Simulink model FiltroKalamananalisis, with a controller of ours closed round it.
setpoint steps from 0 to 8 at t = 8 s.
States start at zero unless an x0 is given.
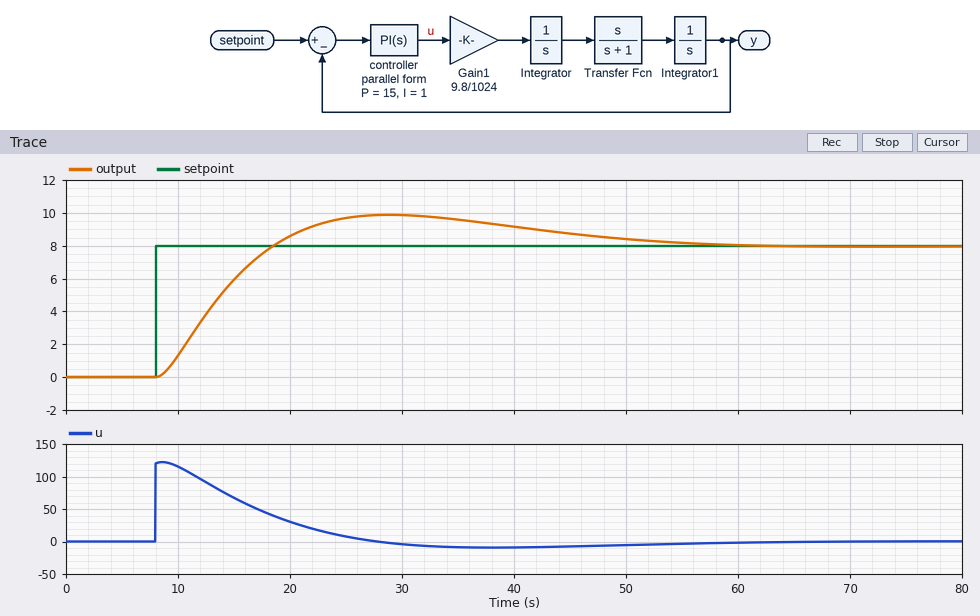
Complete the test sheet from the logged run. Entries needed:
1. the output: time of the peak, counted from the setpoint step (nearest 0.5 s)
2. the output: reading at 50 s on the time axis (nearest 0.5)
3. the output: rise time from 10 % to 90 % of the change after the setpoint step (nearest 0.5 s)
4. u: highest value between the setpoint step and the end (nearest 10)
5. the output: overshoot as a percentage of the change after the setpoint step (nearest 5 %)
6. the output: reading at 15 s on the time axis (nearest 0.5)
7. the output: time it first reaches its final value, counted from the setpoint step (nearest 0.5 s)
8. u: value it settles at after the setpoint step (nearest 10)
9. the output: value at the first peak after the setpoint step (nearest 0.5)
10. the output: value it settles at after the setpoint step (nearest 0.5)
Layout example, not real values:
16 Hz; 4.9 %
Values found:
21.0 s; 8.5; 7.5 s; 120; 25 %; 6.0; 10.5 s; 0; 10.0; 8.0
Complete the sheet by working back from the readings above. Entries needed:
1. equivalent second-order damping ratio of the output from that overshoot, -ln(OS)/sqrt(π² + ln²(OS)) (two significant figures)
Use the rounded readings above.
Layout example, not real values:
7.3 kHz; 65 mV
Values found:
0.40
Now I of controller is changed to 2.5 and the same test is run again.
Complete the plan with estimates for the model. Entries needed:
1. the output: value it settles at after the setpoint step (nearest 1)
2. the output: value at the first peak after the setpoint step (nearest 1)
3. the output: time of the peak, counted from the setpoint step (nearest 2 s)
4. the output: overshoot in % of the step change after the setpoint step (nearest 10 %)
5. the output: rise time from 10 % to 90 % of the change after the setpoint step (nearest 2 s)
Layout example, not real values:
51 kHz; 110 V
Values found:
8; 11; 16 s; 40 %; 6 s
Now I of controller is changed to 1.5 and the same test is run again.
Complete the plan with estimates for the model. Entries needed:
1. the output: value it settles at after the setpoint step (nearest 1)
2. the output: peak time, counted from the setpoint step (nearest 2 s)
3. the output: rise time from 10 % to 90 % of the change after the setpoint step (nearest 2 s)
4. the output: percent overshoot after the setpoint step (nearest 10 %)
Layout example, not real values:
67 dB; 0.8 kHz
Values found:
8; 18 s; 6 s; 30 %
